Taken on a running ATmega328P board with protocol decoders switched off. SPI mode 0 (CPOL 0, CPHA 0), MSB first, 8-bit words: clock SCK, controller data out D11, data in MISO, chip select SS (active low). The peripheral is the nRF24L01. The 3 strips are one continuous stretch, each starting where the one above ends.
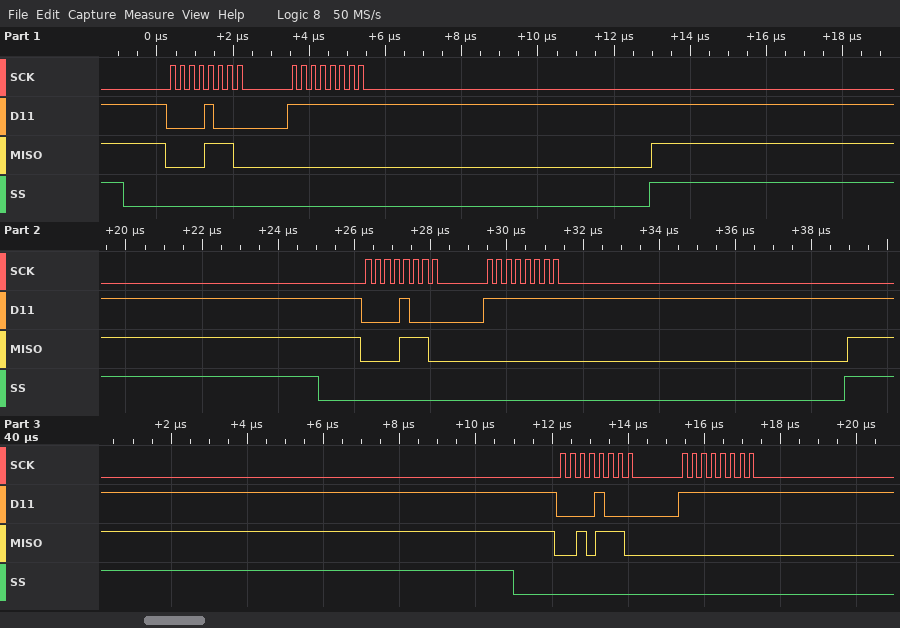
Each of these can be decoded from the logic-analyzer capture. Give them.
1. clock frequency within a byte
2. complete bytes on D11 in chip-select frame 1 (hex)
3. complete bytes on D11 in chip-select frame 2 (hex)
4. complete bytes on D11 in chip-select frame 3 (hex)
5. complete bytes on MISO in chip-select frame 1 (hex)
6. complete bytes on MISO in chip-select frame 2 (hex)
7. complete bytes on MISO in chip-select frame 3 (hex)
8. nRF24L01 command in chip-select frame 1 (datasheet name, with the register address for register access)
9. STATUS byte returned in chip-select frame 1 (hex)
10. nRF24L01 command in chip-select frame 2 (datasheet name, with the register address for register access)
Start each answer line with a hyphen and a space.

- 4 MHz
- 08 FF
- 08 FF
- 08 FF
- 0E 00
- 0E 00
- 2E 00
- R_REGISTER 0x08
- 0x0E
- R_REGISTER 0x08
